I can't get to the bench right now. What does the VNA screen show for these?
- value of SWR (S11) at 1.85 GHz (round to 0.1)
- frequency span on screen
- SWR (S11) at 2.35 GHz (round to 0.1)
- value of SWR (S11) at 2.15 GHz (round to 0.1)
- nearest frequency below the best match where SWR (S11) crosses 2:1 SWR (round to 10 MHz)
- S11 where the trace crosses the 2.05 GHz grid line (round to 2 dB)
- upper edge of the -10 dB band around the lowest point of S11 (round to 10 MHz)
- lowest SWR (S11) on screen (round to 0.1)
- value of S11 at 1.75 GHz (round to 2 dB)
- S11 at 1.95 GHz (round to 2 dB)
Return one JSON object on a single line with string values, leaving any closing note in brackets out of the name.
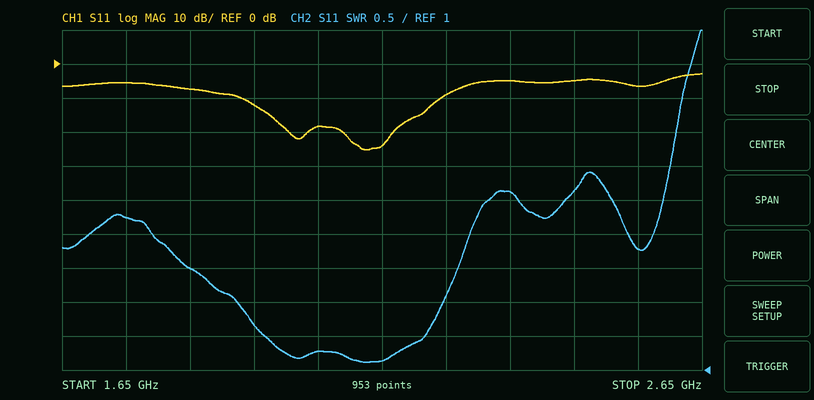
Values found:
{"value of SWR (S11) at 1.85 GHz": "2.5", "frequency span on screen": "1 GHz", "SWR (S11) at 2.35 GHz": "3.6", "value of SWR (S11) at 2.15 GHz": "1.1", "nearest frequency below the best match where SWR (S11) crosses 2:1 SWR": "1.92 GHz", "S11 where the trace crosses the 2.05 GHz grid line": "-18 dB", "upper edge of the -10 dB band around the lowest point of S11": "2.24 GHz", "lowest SWR (S11) on screen": "1.1", "value of S11 at 1.75 GHz": "-6 dB", "S11 at 1.95 GHz": "-12 dB"}
